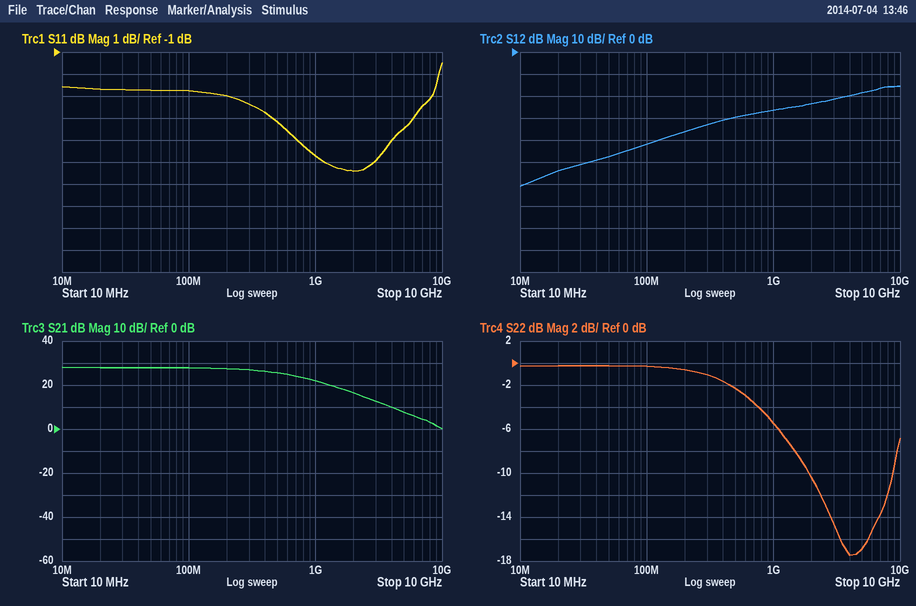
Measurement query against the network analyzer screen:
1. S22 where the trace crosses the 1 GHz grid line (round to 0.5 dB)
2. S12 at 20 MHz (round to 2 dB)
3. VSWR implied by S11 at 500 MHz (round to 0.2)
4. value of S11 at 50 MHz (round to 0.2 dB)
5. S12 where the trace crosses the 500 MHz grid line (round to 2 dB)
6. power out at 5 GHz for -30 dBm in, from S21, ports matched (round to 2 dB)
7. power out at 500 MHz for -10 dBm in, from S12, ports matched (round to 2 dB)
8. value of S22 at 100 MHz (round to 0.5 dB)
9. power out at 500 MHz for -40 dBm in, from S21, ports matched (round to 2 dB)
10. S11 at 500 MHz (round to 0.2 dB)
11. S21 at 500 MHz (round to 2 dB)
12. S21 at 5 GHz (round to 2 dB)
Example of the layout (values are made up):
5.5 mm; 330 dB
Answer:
-5.5 dB; -54 dB; 4.2; -2.8 dB; -30 dB; -22 dBm; -40 dBm; -0.5 dB; -14 dBm; -4.2 dB; 26 dB; 8 dB
